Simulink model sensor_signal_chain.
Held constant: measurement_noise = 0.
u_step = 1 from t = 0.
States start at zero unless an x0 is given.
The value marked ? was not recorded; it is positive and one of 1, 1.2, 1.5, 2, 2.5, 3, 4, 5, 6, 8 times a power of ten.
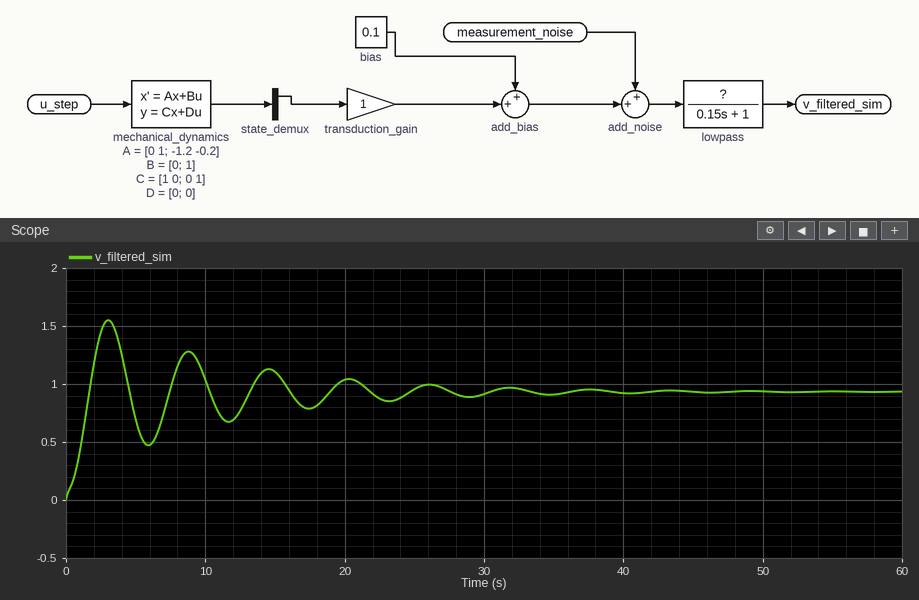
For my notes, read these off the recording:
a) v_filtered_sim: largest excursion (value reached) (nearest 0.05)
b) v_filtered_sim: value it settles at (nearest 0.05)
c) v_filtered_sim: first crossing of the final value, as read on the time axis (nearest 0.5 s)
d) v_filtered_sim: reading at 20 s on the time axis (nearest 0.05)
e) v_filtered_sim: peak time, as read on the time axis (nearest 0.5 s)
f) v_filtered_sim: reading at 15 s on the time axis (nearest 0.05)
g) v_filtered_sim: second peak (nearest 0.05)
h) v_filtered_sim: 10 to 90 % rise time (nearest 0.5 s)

1.55
0.95
1.5 s
1.05
3.0 s
1.10
1.30
1.5 s
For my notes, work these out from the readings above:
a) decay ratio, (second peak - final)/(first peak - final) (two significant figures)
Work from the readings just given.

0.58
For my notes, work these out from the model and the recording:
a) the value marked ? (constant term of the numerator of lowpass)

1
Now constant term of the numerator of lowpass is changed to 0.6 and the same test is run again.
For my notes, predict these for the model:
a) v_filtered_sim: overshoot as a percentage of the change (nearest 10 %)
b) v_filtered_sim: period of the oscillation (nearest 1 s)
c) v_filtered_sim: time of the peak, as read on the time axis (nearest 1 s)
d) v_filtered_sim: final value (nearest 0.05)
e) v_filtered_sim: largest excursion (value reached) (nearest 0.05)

70 %
6 s
3 s
0.55
0.95
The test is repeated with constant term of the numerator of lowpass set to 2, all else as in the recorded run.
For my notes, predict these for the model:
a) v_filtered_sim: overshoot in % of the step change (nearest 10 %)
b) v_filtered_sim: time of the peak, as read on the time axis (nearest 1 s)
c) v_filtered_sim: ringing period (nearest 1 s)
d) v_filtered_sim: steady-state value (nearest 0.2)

70 %
3 s
6 s
1.8
